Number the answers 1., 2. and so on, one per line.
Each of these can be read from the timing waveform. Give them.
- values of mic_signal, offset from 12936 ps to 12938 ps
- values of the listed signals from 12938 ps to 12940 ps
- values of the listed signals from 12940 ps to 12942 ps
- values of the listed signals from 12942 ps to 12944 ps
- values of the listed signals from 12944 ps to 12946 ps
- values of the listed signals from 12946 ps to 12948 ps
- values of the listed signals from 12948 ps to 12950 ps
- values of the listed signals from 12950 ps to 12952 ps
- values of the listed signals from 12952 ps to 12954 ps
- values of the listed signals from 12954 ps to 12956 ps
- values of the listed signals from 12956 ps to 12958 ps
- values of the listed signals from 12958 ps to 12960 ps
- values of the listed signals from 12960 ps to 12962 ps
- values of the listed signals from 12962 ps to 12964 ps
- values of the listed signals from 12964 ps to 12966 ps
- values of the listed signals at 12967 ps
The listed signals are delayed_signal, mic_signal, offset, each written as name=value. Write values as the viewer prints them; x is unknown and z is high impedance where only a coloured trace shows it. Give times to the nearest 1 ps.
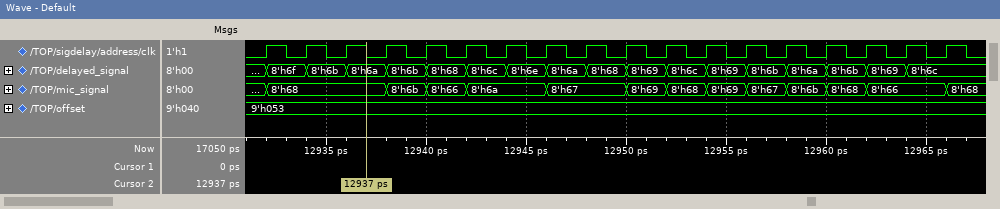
1. mic_signal=8'h68, offset=9'h053
2. delayed_signal=8'h6b, mic_signal=8'h6b, offset=9'h053
3. delayed_signal=8'h68, mic_signal=8'h66, offset=9'h053
4. delayed_signal=8'h6c, mic_signal=8'h6a, offset=9'h053
5. delayed_signal=8'h6e, mic_signal=8'h6a, offset=9'h053
6. delayed_signal=8'h6a, mic_signal=8'h67, offset=9'h053
7. delayed_signal=8'h68, mic_signal=8'h67, offset=9'h053
8. delayed_signal=8'h69, mic_signal=8'h69, offset=9'h053
9. delayed_signal=8'h6c, mic_signal=8'h68, offset=9'h053
10. delayed_signal=8'h69, mic_signal=8'h69, offset=9'h053
11. delayed_signal=8'h6b, mic_signal=8'h67, offset=9'h053
12. delayed_signal=8'h6a, mic_signal=8'h6b, offset=9'h053
13. delayed_signal=8'h6b, mic_signal=8'h68, offset=9'h053
14. delayed_signal=8'h69, mic_signal=8'h66, offset=9'h053
15. delayed_signal=8'h6c, mic_signal=8'h66, offset=9'h053
16. delayed_signal=8'h6c, mic_signal=8'h68, offset=9'h053
